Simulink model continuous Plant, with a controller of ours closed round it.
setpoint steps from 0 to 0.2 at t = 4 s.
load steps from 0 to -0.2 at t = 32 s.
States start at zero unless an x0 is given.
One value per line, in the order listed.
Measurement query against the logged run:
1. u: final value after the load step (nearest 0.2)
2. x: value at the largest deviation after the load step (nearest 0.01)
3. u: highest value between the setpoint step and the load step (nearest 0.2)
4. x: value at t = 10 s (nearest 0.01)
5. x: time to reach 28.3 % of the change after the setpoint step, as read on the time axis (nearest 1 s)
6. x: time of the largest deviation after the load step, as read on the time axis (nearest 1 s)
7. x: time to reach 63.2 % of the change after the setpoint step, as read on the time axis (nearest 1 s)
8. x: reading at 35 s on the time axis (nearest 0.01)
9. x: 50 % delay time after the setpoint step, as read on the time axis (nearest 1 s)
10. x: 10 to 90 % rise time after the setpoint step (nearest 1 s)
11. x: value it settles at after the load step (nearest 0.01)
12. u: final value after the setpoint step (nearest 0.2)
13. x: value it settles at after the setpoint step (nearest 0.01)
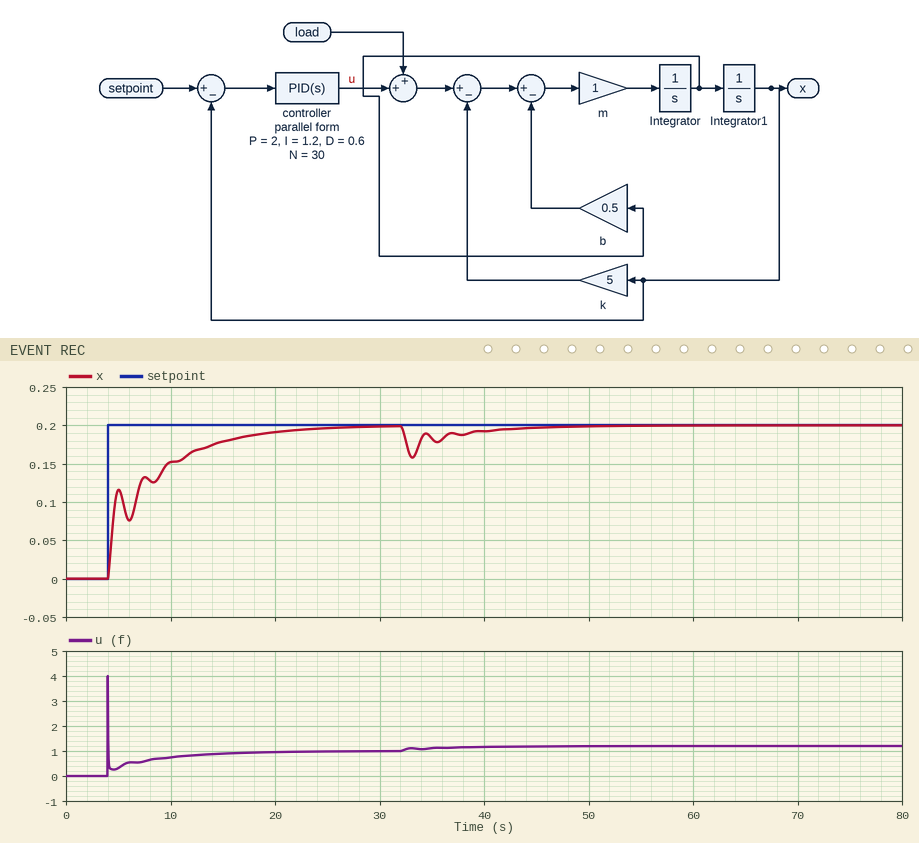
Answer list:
1.2
0.16
4.0
0.15
4 s
33 s
7 s
0.18
5 s
11 s
0.20
1.0
0.20
